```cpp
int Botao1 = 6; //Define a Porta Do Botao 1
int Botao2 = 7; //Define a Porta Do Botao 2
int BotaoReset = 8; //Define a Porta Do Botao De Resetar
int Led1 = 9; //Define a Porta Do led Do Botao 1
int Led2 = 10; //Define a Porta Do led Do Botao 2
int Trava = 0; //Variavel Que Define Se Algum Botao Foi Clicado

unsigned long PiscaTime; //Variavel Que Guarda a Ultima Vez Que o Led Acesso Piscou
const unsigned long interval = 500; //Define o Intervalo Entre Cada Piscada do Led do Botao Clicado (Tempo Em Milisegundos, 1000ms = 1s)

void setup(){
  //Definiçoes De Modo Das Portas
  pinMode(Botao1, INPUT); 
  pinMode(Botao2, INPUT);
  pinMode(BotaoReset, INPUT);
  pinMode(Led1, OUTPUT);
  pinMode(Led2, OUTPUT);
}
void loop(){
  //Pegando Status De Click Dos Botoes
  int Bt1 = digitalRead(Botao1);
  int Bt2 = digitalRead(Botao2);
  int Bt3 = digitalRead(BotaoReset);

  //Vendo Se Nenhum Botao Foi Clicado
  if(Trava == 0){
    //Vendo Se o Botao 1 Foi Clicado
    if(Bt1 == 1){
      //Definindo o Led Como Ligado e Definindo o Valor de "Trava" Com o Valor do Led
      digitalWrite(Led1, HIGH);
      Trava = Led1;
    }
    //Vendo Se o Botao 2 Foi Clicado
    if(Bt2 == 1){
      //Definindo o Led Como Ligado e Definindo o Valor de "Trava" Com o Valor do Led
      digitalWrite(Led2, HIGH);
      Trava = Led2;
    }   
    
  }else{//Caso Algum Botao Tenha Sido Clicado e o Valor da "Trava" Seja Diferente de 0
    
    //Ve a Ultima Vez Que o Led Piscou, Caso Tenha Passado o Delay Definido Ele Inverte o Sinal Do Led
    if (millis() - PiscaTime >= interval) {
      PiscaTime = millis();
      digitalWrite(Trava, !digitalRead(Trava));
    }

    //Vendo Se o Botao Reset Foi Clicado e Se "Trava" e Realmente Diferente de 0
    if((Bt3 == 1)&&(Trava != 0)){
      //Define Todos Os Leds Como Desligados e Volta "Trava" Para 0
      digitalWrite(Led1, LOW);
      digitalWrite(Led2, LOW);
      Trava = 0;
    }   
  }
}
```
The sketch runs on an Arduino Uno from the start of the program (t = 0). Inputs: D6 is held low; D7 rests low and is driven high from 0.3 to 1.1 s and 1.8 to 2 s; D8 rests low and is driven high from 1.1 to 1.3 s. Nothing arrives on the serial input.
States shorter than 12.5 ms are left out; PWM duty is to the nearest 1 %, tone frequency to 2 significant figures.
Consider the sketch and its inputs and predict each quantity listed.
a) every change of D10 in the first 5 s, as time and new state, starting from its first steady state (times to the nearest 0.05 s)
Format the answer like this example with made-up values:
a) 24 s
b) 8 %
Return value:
a) 0 s low; 0.3 s high; 0.5 s low; 1 s high; 1.1 s low; 2.3 s high; 2.8 s low; 3.3 s high; 3.8 s low; 4.3 s high; 4.8 s low
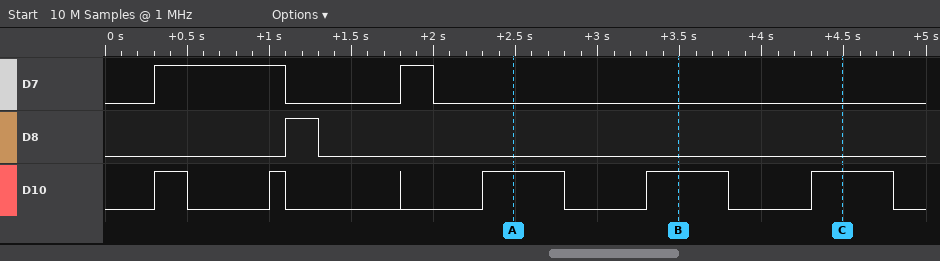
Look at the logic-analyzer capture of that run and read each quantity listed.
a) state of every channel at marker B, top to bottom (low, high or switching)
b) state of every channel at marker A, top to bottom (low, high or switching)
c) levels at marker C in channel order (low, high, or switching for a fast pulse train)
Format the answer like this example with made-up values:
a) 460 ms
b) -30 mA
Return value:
a) D7 low, D8 low, D10 high
b) D7 low, D8 low, D10 high
c) D7 low, D8 low, D10 high
